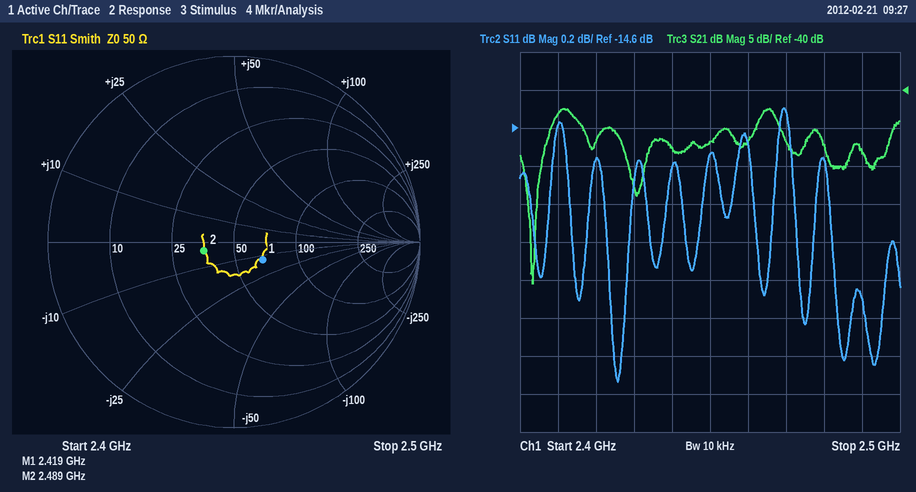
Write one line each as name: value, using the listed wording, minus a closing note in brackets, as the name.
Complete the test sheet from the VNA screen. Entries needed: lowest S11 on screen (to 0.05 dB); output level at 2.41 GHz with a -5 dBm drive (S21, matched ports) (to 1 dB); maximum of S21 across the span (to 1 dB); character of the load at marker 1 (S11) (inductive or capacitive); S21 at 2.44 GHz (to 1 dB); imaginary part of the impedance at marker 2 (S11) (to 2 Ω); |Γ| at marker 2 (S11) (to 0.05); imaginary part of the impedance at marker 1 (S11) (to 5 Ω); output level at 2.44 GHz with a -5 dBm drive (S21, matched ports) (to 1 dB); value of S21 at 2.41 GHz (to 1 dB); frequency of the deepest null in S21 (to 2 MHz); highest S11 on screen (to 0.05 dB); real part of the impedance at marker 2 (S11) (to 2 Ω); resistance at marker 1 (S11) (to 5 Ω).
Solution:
lowest S11 on screen: -15.95 dB
output level at 2.41 GHz with a -5 dBm drive (S21, matched ports): -48 dBm
maximum of S21 across the span: -42 dB
character of the load at marker 1 (S11): capacitive
S21 at 2.44 GHz: -48 dB
imaginary part of the impedance at marker 2 (S11): -4 Ω
|Γ| at marker 2 (S11): 0.15
imaginary part of the impedance at marker 1 (S11): -15 Ω
output level at 2.44 GHz with a -5 dBm drive (S21, matched ports): -53 dBm
value of S21 at 2.41 GHz: -43 dB
frequency of the deepest null in S21: 2.404 GHz
highest S11 on screen: -14.50 dB
real part of the impedance at marker 2 (S11): 36 Ω
resistance at marker 1 (S11): 65 Ω
